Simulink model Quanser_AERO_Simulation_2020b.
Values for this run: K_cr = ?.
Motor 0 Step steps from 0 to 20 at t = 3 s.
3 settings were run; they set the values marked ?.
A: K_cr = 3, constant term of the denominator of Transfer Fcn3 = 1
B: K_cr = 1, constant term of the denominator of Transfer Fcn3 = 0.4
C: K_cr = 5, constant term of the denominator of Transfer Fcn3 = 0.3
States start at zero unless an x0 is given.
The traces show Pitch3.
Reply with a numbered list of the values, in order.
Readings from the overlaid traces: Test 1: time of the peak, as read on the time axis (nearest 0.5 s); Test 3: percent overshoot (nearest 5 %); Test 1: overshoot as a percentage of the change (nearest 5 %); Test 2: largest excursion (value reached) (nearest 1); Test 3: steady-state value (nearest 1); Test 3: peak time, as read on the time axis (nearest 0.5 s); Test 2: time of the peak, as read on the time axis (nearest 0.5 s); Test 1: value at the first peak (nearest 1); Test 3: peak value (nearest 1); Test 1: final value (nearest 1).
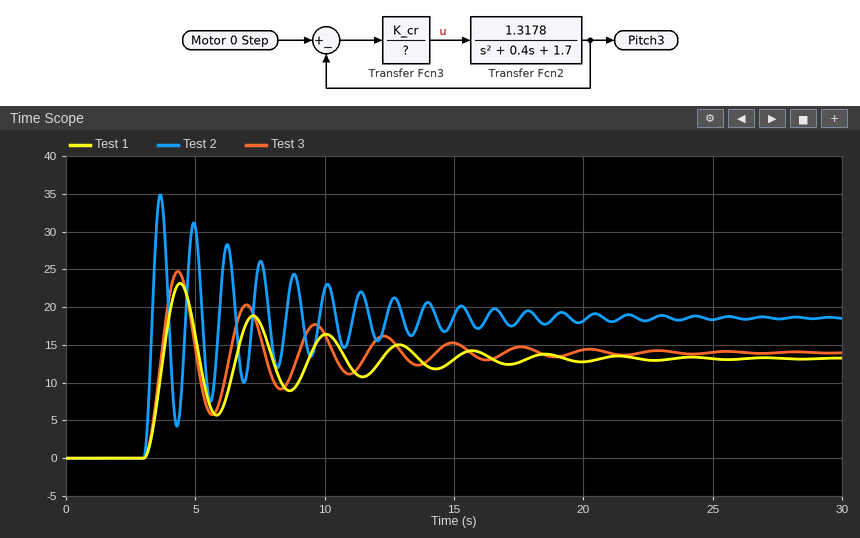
1. 4.5 s
2. 75 %
3. 75 %
4. 35
5. 14
6. 4.5 s
7. 3.5 s
8. 23
9. 25
10. 13
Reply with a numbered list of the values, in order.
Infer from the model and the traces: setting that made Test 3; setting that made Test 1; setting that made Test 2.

1. A
2. B
3. C
